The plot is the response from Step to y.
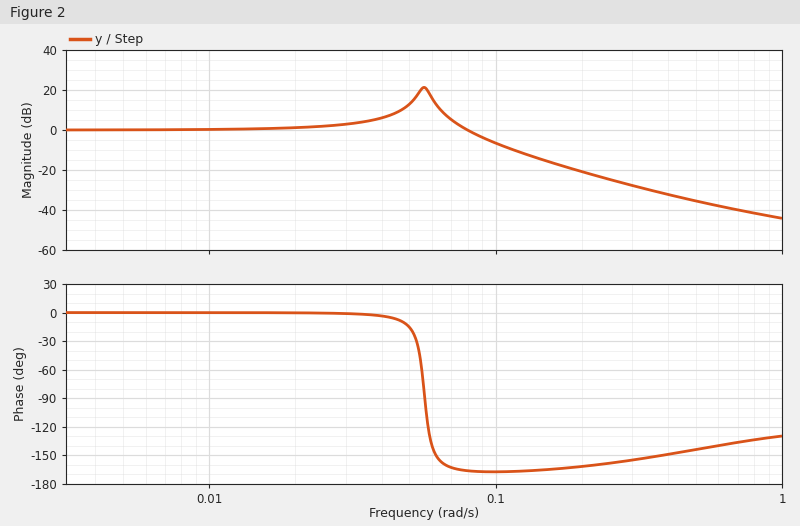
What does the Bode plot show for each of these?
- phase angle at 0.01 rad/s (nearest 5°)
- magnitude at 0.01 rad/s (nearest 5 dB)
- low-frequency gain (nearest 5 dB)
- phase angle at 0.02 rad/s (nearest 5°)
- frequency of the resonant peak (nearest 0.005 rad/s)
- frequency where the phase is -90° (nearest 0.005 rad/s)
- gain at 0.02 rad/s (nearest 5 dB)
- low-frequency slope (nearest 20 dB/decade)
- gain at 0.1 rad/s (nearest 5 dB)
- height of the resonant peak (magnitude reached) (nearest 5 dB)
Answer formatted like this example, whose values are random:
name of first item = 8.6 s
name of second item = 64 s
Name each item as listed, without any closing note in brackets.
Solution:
phase angle at 0.01 rad/s = 0°
magnitude at 0.01 rad/s = 0 dB
low-frequency gain = 0 dB
phase angle at 0.02 rad/s = 0°
frequency of the resonant peak = 0.055 rad/s
frequency where the phase is -90° = 0.055 rad/s
gain at 0.02 rad/s = 0 dB
low-frequency slope = 0 dB/decade
gain at 0.1 rad/s = -5 dB
height of the resonant peak (magnitude reached) = 20 dB
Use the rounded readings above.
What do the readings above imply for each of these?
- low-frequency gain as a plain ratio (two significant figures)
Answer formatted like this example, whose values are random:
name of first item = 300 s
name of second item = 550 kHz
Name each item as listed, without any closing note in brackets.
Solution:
low-frequency gain as a plain ratio = 1.0
